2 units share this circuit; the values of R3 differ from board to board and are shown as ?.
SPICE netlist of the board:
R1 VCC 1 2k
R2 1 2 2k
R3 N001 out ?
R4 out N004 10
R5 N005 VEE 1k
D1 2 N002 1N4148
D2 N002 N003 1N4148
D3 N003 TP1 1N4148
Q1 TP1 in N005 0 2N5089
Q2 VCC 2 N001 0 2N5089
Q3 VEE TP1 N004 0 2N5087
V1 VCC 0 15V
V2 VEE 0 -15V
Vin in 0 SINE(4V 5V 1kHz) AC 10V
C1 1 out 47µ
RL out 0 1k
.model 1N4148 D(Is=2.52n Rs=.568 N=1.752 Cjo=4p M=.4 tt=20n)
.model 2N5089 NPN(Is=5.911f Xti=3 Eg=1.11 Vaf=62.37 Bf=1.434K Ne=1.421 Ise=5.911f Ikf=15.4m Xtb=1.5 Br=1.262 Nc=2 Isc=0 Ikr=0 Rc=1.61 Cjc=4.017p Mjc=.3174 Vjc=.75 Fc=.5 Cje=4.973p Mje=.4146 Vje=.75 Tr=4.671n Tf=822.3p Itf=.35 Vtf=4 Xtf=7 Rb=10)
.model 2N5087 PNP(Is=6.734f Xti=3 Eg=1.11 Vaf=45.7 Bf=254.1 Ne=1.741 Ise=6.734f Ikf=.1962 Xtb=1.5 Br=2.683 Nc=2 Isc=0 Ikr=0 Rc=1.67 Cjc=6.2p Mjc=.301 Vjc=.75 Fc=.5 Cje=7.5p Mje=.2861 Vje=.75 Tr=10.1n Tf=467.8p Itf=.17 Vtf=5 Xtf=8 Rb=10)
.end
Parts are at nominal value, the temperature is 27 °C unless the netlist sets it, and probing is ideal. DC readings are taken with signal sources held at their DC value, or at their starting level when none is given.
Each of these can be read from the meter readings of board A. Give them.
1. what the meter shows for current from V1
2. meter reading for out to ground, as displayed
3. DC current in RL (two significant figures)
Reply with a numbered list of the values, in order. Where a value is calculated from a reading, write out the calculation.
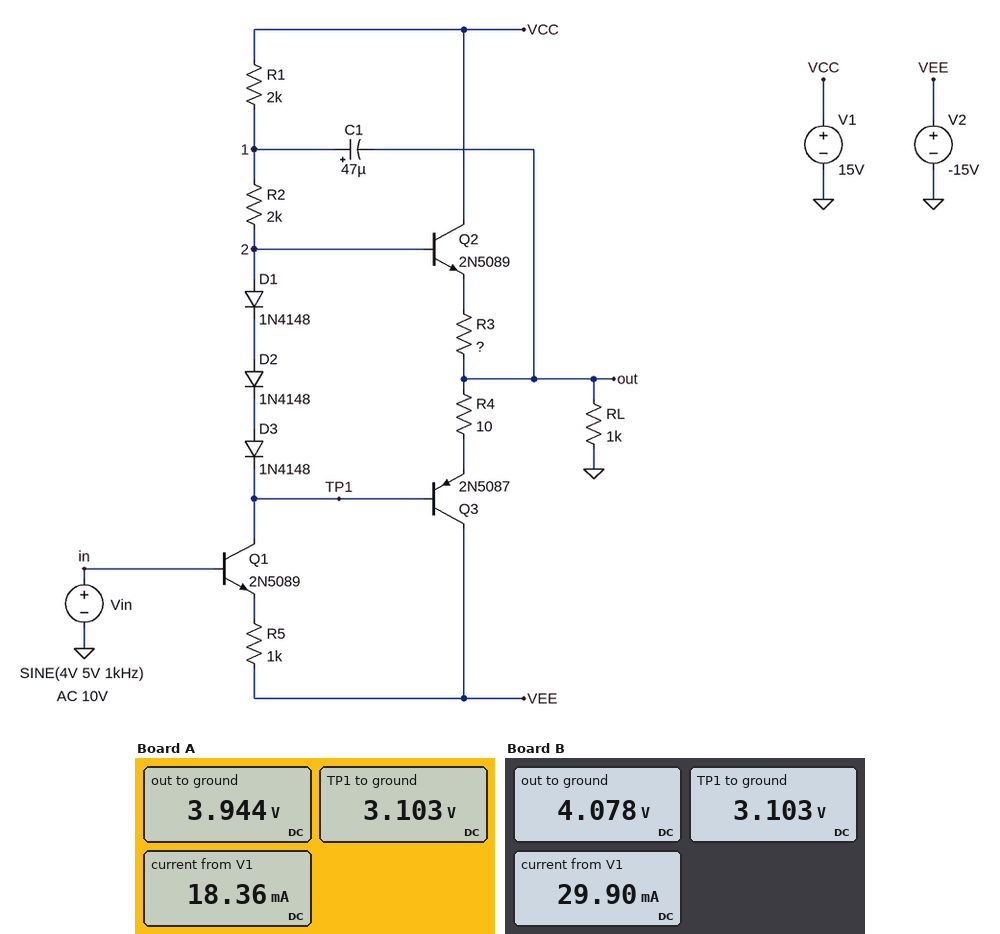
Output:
1. 18.36 mA
2. 3.944 V
3. (3.944 V) / 1 kΩ = 3.9 mA
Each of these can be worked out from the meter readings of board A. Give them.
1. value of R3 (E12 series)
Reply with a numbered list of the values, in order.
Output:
1. 18 Ω
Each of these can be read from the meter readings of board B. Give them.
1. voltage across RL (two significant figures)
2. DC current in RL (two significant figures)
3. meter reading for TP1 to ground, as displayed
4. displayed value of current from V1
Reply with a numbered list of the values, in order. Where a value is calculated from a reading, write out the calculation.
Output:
1. 4.078 V = 4.1 V
2. (4.078 V) / 1 kΩ = 4.1 mA
3. 3.103 V
4. 29.90 mA
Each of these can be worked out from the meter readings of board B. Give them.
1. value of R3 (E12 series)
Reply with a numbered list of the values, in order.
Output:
1. 4.7 Ω
